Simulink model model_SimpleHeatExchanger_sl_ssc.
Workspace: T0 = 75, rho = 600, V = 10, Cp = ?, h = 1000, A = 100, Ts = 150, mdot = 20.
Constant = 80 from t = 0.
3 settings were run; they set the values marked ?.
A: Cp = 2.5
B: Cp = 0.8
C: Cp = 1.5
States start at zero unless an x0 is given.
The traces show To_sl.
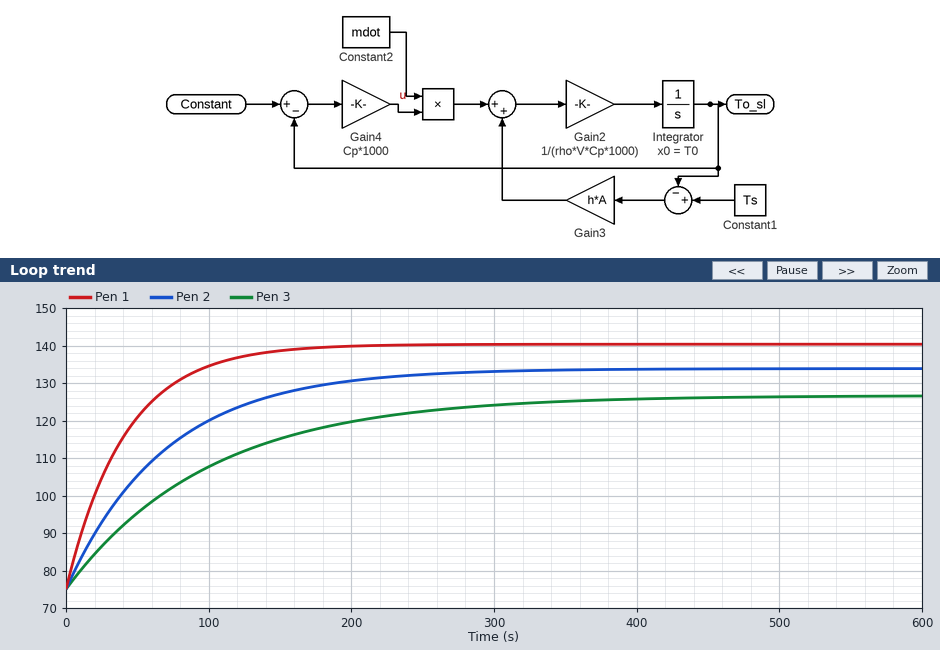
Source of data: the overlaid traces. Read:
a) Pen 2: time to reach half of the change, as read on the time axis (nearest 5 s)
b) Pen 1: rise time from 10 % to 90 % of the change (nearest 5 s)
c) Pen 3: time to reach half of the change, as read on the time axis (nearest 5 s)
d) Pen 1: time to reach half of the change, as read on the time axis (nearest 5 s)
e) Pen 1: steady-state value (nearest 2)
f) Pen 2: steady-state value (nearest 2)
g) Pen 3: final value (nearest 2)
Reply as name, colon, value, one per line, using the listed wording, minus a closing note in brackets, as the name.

Pen 2: time to reach half of the change, as read on the time axis: 50 s
Pen 1: rise time from 10 % to 90 % of the change: 90 s
Pen 3: time to reach half of the change, as read on the time axis: 70 s
Pen 1: time to reach half of the change, as read on the time axis: 30 s
Pen 1: steady-state value: 140
Pen 2: steady-state value: 134
Pen 3: final value: 126
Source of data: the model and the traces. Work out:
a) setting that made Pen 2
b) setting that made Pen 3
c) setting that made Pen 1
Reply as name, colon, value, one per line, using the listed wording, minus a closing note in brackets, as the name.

setting that made Pen 2: C
setting that made Pen 3: A
setting that made Pen 1: B
